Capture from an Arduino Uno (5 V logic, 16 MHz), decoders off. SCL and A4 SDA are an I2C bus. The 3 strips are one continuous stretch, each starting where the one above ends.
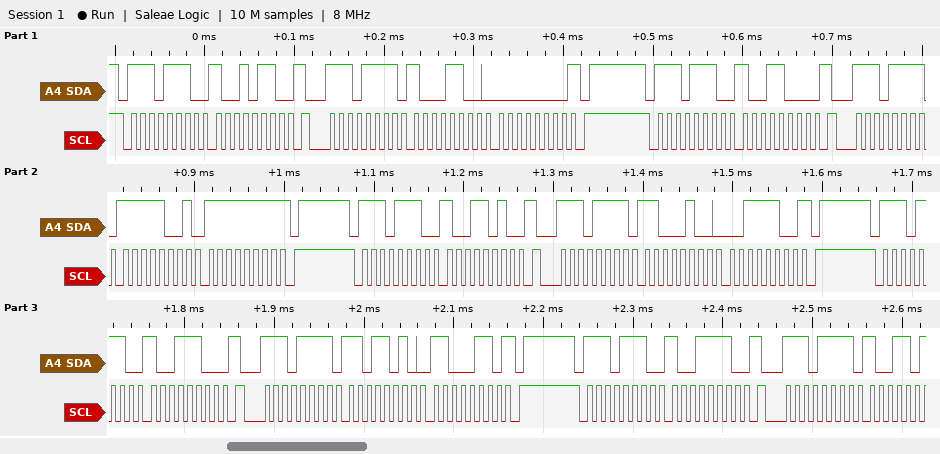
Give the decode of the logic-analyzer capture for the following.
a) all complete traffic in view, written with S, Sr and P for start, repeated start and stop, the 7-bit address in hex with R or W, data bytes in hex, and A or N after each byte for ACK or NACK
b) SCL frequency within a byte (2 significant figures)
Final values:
S 77W A 96 A Sr 77R A 8C A 00 N P S 77W A 98 A Sr 77R A F9 A FF N P S 77W A 9A A Sr 77R A C4 A 3C N P S 77W A 9C A Sr 77R A DA A C6 N P S 77W A 9E A Sr 77R A
100 kHz
